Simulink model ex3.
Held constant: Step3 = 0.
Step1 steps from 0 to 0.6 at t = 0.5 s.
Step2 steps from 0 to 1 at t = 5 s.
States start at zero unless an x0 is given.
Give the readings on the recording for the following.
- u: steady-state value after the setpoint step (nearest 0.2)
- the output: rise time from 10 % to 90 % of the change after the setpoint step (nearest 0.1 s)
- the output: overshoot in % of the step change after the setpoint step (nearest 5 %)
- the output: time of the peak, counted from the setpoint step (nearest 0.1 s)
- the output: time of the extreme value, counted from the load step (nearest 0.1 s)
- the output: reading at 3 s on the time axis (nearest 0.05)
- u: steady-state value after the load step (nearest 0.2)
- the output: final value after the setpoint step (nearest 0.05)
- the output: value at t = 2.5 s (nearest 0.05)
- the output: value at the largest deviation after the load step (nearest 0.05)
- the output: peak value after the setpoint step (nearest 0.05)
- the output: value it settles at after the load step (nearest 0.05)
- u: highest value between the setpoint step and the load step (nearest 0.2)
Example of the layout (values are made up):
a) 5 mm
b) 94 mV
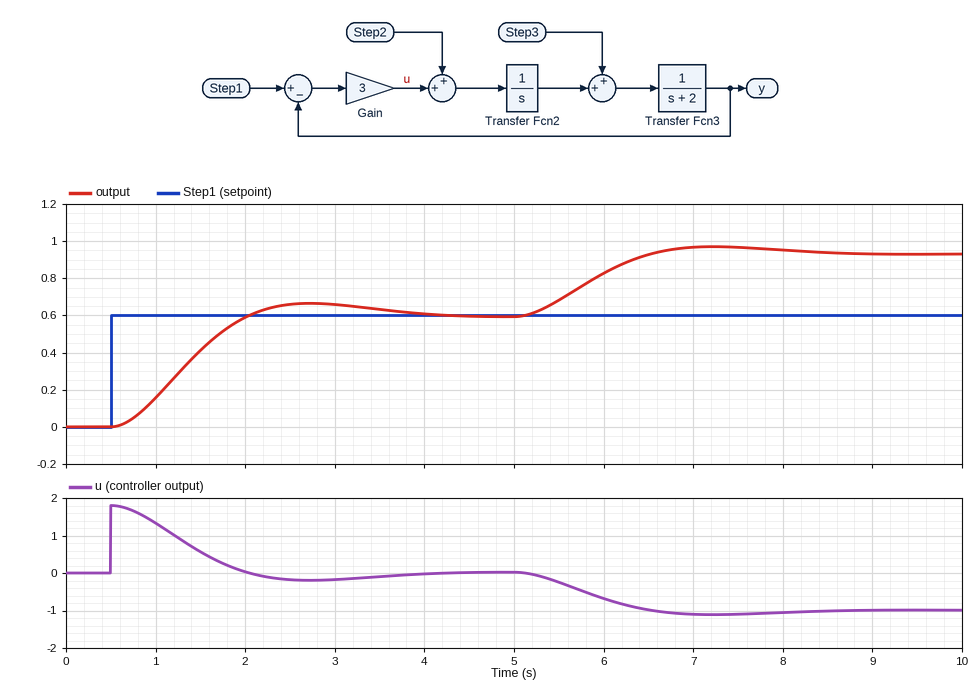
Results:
a) 0.0
b) 1.0 s
c) 10 %
d) 2.2 s
e) 2.2 s
f) 0.65
g) -1.0
h) 0.60
i) 0.65
j) 0.95
k) 0.65
l) 0.95
m) 1.8
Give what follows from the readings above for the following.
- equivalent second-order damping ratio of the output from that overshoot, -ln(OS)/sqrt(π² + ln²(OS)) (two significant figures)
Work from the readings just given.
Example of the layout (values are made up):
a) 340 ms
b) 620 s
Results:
a) 0.59
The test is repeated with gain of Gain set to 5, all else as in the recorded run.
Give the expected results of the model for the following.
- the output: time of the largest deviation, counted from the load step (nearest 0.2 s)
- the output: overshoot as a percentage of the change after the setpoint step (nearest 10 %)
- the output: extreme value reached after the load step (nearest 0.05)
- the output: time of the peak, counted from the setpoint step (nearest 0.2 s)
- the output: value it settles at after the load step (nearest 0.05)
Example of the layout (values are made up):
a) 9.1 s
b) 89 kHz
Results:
a) 1.6 s
b) 20 %
c) 0.85
d) 1.6 s
e) 0.80
